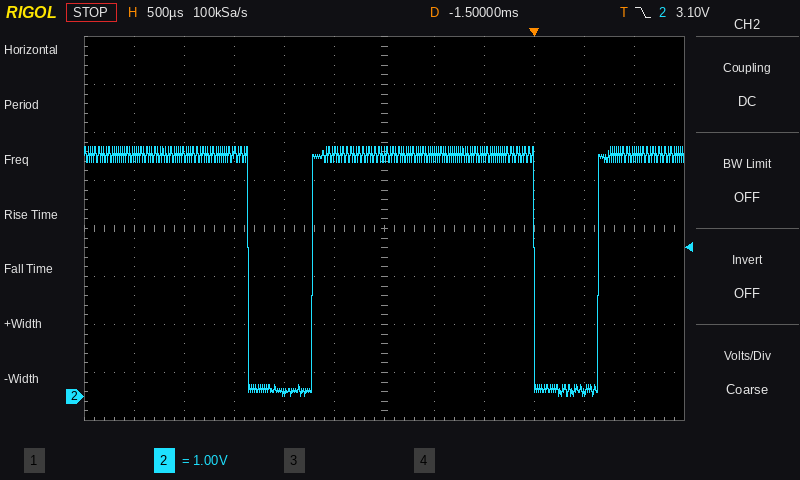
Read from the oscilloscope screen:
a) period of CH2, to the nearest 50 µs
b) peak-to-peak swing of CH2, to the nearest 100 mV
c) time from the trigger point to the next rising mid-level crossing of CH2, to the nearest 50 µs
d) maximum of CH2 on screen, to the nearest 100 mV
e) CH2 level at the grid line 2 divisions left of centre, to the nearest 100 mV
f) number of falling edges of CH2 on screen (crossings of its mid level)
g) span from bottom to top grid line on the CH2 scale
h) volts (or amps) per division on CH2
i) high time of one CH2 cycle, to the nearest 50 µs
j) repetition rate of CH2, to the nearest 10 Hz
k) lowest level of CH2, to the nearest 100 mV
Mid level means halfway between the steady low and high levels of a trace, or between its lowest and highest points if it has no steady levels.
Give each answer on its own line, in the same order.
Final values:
2.85 ms
5.2 V
650 µs
5.2 V
100 mV
2
8 V
1 V
2.20 ms
350 Hz
0.0 V
